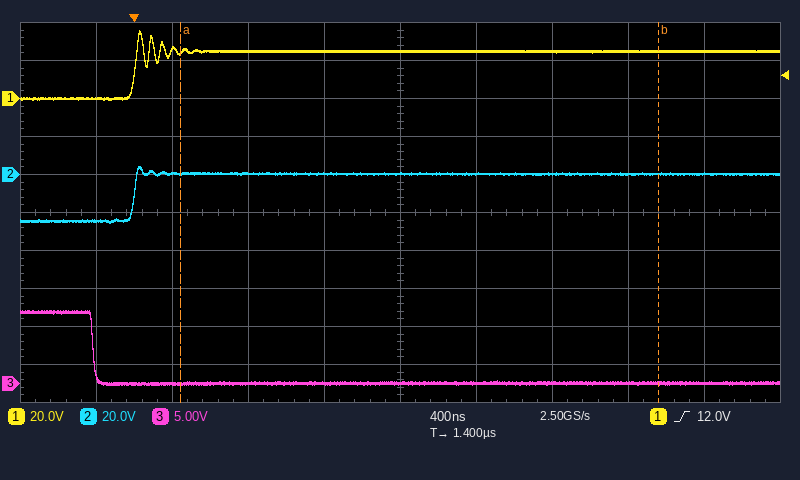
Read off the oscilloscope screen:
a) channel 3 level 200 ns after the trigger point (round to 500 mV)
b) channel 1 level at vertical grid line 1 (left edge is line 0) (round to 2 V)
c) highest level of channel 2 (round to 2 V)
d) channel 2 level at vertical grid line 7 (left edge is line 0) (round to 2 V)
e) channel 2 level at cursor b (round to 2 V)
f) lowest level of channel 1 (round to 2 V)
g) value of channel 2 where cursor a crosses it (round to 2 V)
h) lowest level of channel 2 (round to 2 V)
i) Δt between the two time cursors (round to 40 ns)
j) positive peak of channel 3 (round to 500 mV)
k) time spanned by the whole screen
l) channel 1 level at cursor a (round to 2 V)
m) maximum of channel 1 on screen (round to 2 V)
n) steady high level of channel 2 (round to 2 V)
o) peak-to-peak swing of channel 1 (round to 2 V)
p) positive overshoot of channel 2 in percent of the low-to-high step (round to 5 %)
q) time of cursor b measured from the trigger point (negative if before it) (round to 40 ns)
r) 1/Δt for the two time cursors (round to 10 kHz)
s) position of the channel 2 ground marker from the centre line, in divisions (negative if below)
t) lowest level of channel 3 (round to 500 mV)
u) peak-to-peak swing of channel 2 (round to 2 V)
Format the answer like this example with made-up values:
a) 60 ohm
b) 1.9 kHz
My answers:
a) 0.0 V
b) 0 V
c) 4 V
d) 0 V
e) 0 V
f) 0 V
g) 0 V
h) -26 V
i) 2.52 µs
j) 9.5 V
k) 4 µs
l) 24 V
m) 36 V
n) 0 V
o) 36 V
p) 15 %
q) +2.76 µs
r) 400 kHz
s) +1.0 div
t) 0.0 V
u) 30 V
